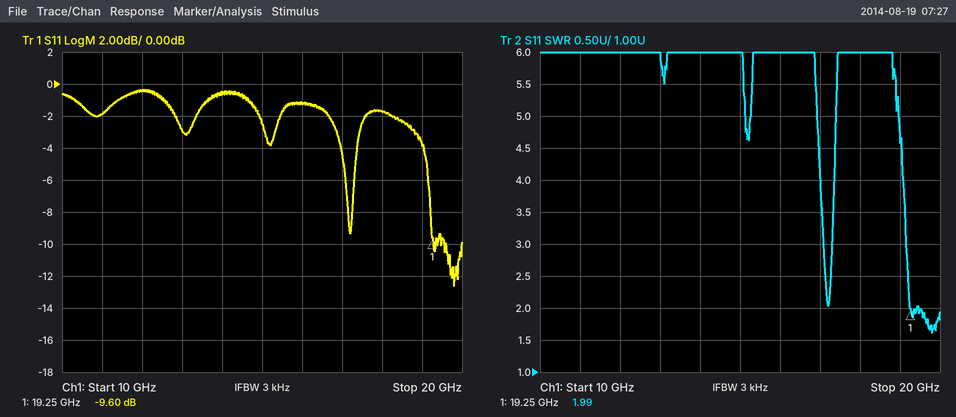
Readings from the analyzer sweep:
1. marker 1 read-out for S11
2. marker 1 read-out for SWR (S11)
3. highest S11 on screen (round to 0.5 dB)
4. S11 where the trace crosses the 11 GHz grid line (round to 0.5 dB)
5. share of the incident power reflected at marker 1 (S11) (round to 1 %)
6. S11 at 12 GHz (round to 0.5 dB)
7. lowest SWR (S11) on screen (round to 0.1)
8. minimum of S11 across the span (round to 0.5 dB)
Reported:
-9.60 dB
1.99
-0.5 dB
-2.0 dB
11 %
-0.5 dB
1.6
-12.5 dB
